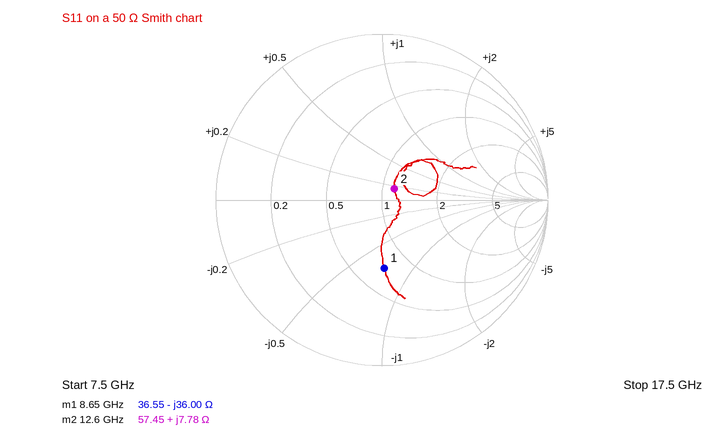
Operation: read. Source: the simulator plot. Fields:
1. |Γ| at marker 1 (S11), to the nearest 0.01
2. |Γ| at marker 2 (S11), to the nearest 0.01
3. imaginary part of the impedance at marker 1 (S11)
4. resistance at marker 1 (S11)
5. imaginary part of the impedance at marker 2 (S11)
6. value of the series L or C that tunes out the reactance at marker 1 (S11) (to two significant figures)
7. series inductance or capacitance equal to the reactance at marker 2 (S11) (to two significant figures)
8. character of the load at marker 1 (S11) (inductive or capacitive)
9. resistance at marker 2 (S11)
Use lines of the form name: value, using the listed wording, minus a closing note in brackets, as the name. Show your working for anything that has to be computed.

|Γ| at marker 1 (S11), to the nearest 0.01: 0.41
|Γ| at marker 2 (S11), to the nearest 0.01: 0.10
imaginary part of the impedance at marker 1: -36.00 Ω
resistance at marker 1: 36.55 Ω
imaginary part of the impedance at marker 2: +7.78 Ω
value of the series L or C that tunes out the reactance at marker 1 (S11): L = 36 Ω/(2π × 8.65 GHz) ≈ 662 pH, so 660 pH to two significant figures
series inductance or capacitance equal to the reactance at marker 2 (S11): L = 7.78 Ω/(2π × 12.6 GHz) ≈ 98 pH
character of the load at marker 1 (S11): capacitive
resistance at marker 2: 57.45 Ω
